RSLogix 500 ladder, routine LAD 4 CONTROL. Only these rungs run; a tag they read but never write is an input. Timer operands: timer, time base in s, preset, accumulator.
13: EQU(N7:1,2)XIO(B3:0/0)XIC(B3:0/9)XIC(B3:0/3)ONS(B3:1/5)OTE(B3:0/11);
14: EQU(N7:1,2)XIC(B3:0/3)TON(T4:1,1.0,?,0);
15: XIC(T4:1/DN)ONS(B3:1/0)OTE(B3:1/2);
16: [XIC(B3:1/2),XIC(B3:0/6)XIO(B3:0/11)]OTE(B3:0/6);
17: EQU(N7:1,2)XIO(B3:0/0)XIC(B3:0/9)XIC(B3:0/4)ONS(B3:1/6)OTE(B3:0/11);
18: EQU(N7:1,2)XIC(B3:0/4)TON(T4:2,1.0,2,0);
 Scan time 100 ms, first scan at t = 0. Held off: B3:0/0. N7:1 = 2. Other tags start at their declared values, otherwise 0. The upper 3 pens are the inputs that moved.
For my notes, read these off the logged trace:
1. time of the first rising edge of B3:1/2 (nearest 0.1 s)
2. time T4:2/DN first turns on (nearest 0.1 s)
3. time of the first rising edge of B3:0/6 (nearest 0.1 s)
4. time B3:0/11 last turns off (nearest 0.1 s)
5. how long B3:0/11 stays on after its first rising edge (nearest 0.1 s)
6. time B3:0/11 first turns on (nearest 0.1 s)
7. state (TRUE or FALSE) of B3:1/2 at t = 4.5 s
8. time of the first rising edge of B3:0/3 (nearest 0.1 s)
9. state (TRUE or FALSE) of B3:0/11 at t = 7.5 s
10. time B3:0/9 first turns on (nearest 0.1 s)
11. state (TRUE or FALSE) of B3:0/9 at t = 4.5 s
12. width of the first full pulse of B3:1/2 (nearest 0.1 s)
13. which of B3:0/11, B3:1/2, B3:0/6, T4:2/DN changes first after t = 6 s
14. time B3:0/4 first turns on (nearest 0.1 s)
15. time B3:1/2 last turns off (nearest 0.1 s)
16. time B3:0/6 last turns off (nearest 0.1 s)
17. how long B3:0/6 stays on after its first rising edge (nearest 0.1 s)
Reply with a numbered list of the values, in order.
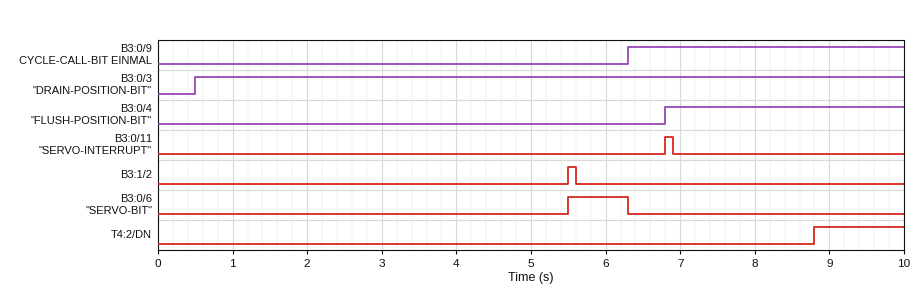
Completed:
1. 5.5 s
2. 8.8 s
3. 5.5 s
4. 6.9 s
5. 0.1 s
6. 6.8 s
7. FALSE
8. 0.5 s
9. FALSE
10. 6.3 s
11. FALSE
12. 0.1 s
13. B3:0/6
14. 6.8 s
15. 5.6 s
16. 6.3 s
17. 0.8 s
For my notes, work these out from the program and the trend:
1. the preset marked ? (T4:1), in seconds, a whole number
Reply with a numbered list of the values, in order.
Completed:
1. 5 s
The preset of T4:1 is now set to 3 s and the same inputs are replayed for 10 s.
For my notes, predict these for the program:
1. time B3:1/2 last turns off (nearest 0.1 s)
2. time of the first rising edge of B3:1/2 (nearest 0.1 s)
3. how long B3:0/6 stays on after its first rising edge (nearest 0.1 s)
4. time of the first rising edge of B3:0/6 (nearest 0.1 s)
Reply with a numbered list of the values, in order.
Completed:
1. 3.6 s
2. 3.5 s
3. 2.8 s
4. 3.5 s
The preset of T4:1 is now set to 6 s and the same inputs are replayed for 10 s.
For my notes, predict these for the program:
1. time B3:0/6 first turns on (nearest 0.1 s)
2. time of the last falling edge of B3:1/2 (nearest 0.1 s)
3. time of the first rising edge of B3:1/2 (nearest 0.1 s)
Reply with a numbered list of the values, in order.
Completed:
1. 6.5 s
2. 6.6 s
3. 6.5 s
